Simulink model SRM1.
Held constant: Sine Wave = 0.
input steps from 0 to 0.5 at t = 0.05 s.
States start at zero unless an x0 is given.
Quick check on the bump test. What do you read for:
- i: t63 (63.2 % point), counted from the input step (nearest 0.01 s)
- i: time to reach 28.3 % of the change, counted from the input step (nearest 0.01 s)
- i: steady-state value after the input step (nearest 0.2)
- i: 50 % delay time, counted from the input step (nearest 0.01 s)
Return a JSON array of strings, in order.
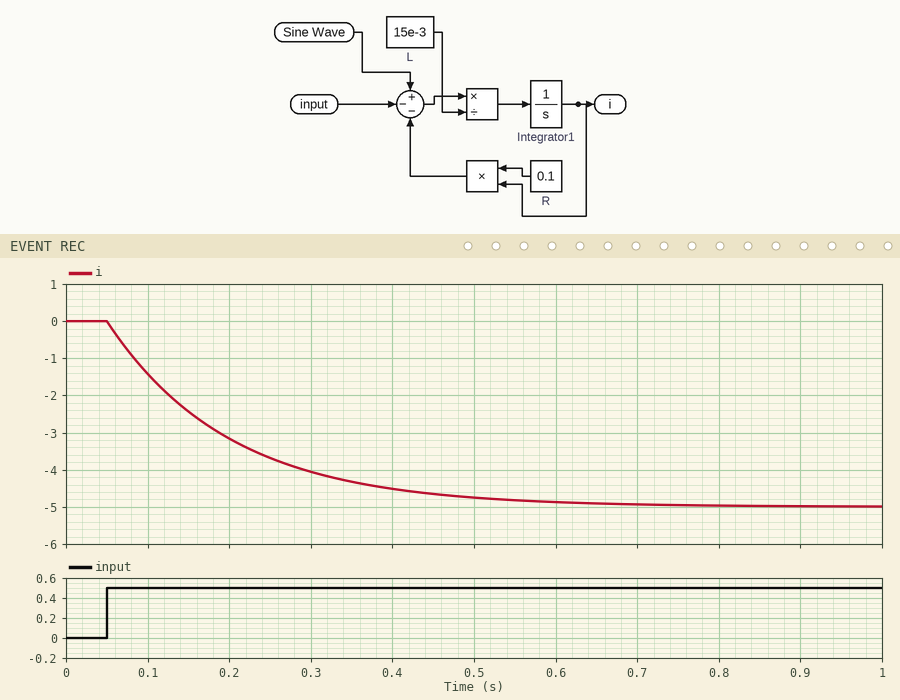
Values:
["0.15 s", "0.05 s", "-5.0", "0.10 s"]
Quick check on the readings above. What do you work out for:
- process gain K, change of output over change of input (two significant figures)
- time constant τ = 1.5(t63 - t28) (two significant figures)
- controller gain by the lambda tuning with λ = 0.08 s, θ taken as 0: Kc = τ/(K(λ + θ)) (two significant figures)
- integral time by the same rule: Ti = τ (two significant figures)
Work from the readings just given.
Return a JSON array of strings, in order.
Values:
["-10", "0.15 s", "-0.19", "0.15 s"]
